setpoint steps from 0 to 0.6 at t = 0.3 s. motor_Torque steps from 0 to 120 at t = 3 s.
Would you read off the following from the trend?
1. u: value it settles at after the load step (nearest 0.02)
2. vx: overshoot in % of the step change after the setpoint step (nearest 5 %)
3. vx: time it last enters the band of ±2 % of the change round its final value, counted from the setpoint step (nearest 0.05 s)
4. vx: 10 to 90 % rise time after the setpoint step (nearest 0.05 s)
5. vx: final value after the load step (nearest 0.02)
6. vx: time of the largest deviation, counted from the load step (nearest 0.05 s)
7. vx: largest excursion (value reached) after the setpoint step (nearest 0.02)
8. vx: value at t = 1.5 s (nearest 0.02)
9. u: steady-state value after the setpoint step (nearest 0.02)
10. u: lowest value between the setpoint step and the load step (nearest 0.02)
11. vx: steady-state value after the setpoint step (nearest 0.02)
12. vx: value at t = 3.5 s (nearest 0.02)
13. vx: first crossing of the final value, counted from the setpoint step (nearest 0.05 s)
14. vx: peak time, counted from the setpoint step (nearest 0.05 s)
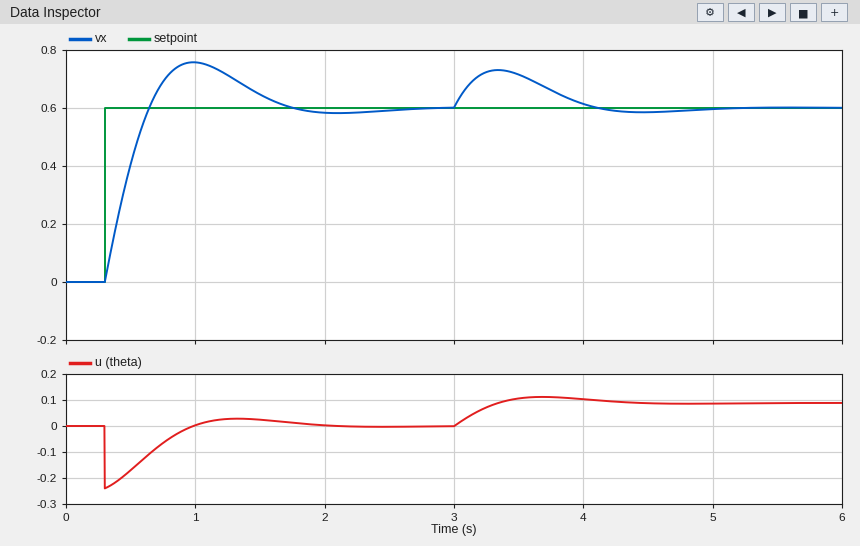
0.08
25 %
2.10 s
0.25 s
0.60
0.35 s
0.76
0.64
0.00
-0.24
0.60
0.72
0.35 s
0.70 s
